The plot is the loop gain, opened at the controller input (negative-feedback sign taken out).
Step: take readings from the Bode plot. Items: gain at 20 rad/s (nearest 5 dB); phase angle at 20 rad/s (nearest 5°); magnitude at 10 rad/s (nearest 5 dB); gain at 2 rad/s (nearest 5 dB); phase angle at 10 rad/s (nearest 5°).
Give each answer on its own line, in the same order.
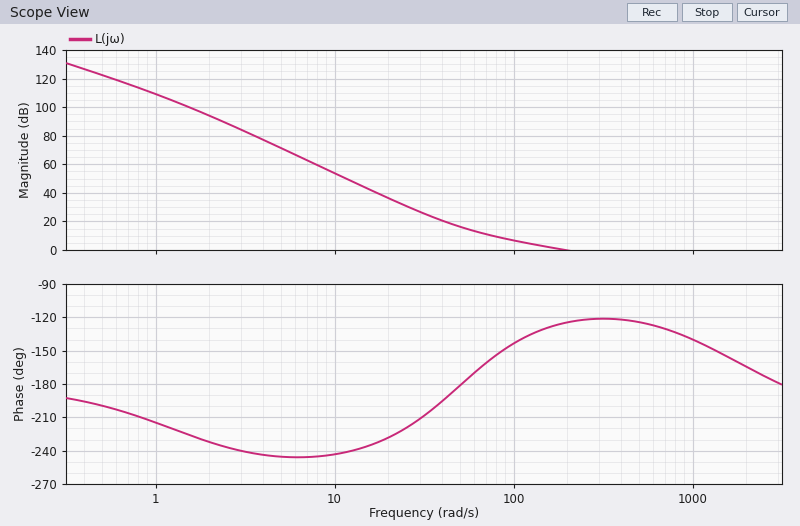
35 dB
-230°
55 dB
95 dB
-245°
